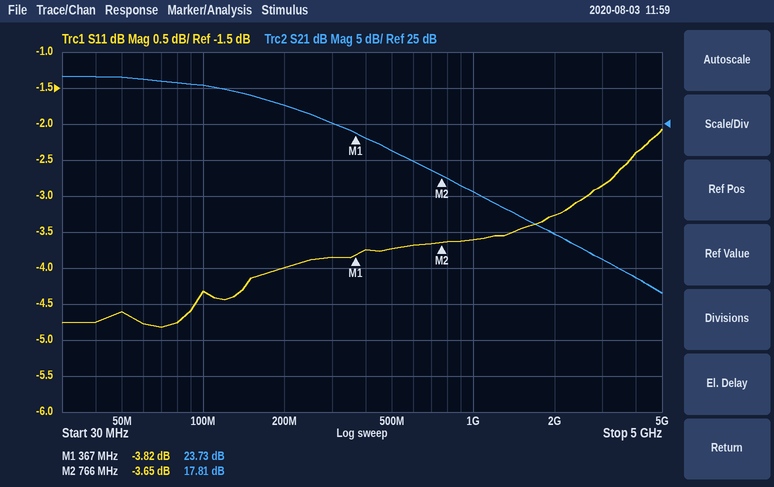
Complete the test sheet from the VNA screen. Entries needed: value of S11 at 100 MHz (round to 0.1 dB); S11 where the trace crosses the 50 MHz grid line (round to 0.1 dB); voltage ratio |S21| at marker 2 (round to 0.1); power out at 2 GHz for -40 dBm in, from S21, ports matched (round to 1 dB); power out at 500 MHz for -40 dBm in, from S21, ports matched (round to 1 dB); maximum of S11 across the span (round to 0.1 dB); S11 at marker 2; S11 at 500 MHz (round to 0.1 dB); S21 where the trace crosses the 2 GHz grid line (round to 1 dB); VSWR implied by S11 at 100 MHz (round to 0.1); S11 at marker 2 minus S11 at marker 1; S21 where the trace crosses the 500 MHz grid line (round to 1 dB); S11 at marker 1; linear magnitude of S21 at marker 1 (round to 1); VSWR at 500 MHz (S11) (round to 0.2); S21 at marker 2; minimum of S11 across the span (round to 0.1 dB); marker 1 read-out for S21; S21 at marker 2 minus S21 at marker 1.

-4.3 dB
-4.6 dB
7.8
-30 dBm
-19 dBm
-2.1 dB
-3.65 dB
-3.7 dB
10 dB
4.1
0.17 dB
21 dB
-3.82 dB
15
4.8
17.81 dB
-4.8 dB
23.73 dB
-5.92 dB
